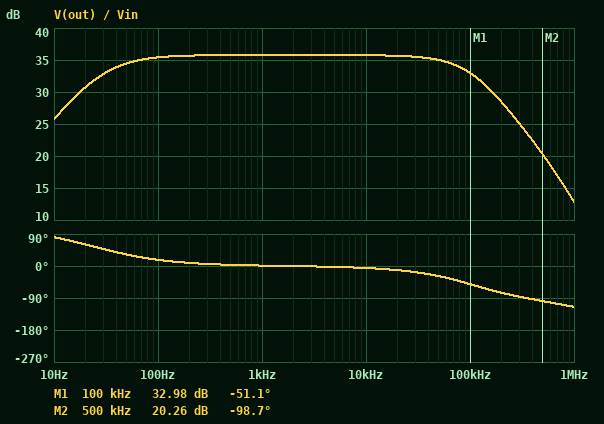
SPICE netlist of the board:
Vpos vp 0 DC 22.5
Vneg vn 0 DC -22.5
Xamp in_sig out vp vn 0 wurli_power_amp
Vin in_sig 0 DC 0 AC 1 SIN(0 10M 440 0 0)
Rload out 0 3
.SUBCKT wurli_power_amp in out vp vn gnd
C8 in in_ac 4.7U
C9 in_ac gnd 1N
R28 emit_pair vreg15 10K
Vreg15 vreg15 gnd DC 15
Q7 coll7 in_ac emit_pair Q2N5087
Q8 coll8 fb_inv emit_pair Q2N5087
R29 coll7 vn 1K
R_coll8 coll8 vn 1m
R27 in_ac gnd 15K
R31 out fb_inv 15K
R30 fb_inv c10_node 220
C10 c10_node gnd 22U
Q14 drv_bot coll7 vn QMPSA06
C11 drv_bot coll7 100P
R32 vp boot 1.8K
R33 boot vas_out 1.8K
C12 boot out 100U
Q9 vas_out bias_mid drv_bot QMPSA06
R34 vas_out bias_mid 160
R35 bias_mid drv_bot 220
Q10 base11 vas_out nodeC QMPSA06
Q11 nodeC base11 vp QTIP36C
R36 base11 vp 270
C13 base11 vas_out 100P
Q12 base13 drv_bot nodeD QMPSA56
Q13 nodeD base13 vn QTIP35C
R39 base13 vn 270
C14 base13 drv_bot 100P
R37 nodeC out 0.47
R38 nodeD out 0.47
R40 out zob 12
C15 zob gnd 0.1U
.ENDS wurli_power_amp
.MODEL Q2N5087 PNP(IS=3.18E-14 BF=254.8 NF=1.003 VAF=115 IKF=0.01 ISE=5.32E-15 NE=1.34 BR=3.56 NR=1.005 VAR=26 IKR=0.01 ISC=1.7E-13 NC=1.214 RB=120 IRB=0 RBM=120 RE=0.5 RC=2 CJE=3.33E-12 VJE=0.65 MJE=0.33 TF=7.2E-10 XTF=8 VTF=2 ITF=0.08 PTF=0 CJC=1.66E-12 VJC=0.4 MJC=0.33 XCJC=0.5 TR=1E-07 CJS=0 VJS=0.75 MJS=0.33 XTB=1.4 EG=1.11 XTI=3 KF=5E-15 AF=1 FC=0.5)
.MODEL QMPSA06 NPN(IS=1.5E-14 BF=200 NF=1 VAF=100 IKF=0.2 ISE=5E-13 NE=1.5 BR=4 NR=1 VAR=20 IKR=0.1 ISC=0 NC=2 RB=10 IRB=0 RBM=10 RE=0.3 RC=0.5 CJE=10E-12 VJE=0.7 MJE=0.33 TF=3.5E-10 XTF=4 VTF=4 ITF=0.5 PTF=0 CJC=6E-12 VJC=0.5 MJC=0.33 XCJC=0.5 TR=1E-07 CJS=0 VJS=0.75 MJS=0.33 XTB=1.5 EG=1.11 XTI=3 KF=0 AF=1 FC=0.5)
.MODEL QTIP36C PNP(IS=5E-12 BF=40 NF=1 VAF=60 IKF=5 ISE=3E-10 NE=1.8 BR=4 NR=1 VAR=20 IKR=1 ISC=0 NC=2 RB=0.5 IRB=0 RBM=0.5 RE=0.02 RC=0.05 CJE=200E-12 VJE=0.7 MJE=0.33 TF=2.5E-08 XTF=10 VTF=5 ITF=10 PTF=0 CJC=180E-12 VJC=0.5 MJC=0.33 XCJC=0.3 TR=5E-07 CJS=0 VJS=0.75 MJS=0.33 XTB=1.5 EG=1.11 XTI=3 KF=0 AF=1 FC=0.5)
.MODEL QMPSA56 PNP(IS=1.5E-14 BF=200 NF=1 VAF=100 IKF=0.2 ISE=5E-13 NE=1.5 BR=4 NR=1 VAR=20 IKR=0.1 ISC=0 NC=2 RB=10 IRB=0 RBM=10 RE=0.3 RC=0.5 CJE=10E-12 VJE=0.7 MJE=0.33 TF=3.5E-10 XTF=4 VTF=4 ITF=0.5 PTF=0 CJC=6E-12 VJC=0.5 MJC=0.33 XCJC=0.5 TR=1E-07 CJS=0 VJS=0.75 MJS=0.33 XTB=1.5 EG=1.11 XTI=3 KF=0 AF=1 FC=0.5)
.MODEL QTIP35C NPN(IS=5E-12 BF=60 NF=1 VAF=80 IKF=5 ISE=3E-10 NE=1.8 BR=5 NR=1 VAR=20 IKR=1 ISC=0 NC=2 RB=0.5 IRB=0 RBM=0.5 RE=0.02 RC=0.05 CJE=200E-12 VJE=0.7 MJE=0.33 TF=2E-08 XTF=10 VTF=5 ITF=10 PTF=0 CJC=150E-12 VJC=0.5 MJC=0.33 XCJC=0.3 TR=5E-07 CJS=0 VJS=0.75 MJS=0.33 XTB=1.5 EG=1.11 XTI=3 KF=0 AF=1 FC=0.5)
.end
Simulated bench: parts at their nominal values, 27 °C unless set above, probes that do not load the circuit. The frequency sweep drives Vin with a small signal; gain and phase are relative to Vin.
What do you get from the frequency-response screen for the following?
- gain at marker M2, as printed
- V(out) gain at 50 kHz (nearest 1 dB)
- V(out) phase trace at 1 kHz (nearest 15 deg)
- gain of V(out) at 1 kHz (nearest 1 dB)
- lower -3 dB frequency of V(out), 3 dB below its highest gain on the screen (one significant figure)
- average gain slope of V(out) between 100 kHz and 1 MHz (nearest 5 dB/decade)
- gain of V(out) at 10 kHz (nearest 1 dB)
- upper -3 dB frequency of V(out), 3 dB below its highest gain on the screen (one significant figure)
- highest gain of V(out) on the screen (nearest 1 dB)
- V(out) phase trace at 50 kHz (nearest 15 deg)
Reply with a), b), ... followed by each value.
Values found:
a) 20.26 dB
b) 35 dB
c) 0 deg
d) 36 dB
e) 30 Hz
f) -20 dB/decade
g) 36 dB
h) 100 kHz
i) 36 dB
j) -30 deg
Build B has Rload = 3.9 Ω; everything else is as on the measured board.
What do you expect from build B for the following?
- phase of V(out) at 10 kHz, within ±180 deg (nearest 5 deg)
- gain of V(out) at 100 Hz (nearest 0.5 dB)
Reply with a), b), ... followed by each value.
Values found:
a) -10 deg
b) 34.5 dB
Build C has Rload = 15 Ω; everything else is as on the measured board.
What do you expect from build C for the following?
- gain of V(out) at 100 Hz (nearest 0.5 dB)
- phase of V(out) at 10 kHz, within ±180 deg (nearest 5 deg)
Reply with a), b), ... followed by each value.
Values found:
a) 35.0 dB
b) -10 deg
